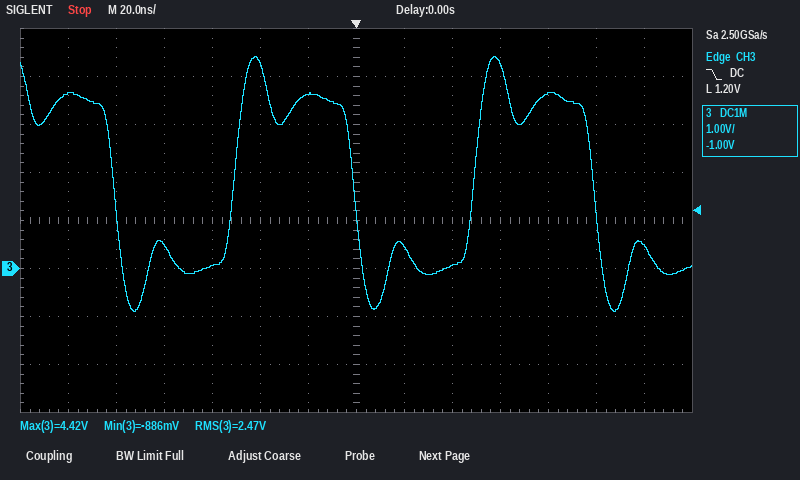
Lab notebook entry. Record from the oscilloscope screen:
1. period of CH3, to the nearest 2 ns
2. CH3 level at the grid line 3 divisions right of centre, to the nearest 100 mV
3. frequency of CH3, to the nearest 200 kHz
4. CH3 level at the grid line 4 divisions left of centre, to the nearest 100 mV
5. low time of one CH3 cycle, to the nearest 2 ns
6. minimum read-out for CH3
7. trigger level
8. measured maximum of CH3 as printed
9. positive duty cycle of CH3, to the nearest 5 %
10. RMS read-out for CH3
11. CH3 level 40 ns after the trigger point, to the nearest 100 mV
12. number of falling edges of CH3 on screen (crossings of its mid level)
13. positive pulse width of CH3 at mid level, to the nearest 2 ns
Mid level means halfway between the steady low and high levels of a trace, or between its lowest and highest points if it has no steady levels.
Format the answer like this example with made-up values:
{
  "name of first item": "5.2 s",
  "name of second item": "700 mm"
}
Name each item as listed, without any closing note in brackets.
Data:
{
  "period of CH3, to the nearest 2 ns": "100 ns",
  "CH3 level at the grid line 3 divisions right of centre, to the nearest 100 mV": "4.3 V",
  "frequency of CH3, to the nearest 200 kHz": "10.0 MHz",
  "CH3 level at the grid line 4 divisions left of centre, to the nearest 100 mV": "500 mV",
  "low time of one CH3 cycle, to the nearest 2 ns": "50 ns",
  "minimum read-out for CH3": "-886 mV",
  "trigger level": "1.20 V",
  "measured maximum of CH3 as printed": "4.42 V",
  "positive duty cycle of CH3, to the nearest 5 %": "50 %",
  "RMS read-out for CH3": "2.47 V",
  "CH3 level 40 ns after the trigger point, to the nearest 100 mV": "100 mV",
  "number of falling edges of CH3 on screen": "3",
  "positive pulse width of CH3 at mid level, to the nearest 2 ns": "50 ns"
}
